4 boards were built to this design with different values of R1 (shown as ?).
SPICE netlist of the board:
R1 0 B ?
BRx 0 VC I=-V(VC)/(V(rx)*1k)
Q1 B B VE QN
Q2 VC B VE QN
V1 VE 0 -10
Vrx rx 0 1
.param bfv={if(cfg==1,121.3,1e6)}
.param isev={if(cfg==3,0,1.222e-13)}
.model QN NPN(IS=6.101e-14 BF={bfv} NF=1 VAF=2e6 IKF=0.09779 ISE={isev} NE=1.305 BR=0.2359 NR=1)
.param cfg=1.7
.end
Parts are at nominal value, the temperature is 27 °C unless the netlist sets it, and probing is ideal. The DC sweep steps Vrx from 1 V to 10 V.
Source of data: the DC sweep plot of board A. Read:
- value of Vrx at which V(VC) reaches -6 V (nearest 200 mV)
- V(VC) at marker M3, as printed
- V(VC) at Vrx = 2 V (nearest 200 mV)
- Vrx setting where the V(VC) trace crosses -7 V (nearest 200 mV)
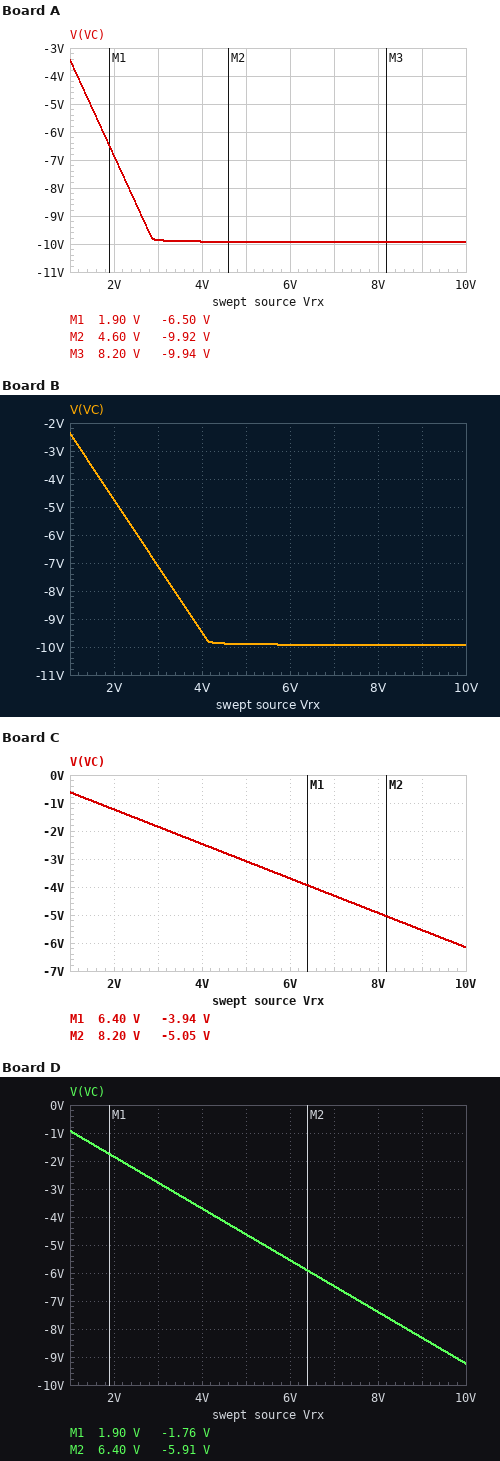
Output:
1.8 V
-9.94 V
-6.8 V
2.0 V
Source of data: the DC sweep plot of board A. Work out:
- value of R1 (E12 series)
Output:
2.7 kΩ
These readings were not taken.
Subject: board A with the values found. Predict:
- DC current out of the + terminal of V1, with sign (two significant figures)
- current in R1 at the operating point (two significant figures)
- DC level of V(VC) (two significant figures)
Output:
-6.9 mA
3.5 mA
-3.4 V
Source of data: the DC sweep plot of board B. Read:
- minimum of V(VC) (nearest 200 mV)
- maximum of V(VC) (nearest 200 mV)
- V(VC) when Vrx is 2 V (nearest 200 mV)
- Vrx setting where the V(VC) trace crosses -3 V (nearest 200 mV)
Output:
-10.0 V
-2.4 V
-4.8 V
1.2 V
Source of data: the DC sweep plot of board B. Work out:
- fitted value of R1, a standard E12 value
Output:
3.9 kΩ
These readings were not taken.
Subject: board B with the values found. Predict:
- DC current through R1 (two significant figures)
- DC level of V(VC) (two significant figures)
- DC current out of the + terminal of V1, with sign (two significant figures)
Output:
2.4 mA
-2.4 V
-4.8 mA
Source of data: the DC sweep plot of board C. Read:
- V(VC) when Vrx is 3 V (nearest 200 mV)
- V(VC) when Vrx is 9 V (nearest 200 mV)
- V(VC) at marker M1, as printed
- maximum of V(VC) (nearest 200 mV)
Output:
-1.8 V
-5.6 V
-3.94 V
-600 mV
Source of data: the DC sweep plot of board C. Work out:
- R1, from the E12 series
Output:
15 kΩ
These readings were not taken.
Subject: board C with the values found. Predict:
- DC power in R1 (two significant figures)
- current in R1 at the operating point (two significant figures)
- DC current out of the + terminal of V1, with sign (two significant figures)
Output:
5.9 mW
630 µA
-1.2 mA
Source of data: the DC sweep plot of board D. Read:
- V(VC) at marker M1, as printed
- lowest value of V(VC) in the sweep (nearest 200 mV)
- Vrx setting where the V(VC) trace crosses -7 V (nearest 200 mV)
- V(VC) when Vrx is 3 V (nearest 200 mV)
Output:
-1.76 V
-9.2 V
7.6 V
-2.8 V
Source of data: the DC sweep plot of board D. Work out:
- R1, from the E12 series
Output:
10 kΩ
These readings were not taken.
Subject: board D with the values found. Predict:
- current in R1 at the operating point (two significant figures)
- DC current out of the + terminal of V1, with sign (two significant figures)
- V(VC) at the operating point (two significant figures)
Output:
940 µA
-1.9 mA
-920 mV
